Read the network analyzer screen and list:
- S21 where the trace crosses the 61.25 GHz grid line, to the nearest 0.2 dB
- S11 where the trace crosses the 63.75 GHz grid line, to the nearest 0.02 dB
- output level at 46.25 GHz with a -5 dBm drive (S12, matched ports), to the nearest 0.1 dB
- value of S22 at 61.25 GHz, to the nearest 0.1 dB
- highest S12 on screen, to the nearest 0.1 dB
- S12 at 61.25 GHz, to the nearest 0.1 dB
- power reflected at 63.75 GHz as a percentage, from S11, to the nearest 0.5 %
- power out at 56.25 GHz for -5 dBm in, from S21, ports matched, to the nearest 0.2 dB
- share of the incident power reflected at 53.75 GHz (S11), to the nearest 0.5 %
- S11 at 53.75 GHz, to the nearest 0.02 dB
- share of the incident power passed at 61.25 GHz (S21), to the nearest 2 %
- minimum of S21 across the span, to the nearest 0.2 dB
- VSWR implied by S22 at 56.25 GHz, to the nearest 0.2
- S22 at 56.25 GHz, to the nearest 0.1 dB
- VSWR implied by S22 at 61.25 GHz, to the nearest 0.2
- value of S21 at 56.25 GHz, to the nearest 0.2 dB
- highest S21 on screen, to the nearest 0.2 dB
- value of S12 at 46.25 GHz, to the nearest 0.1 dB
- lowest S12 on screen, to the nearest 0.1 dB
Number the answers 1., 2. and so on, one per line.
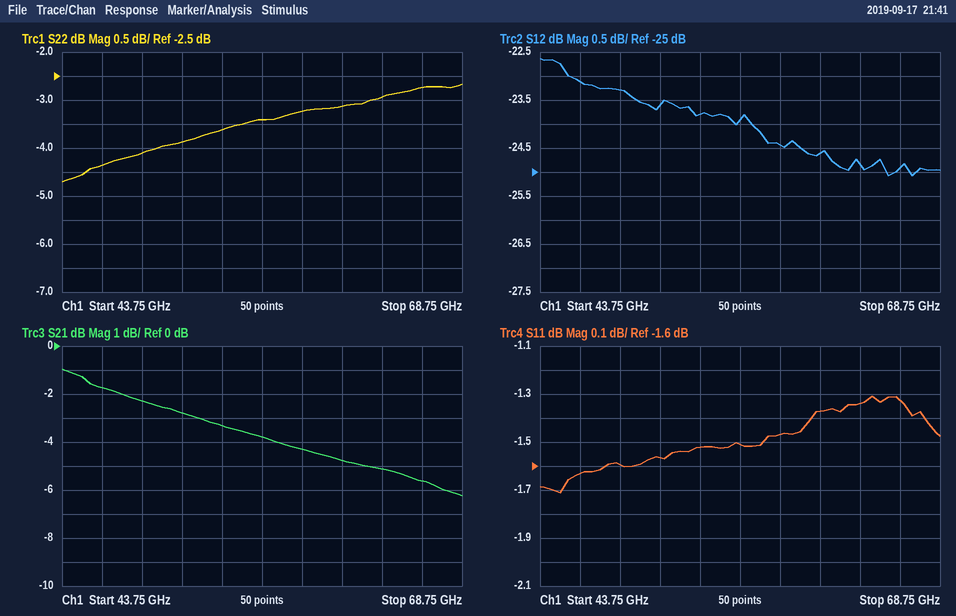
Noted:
1. -4.8 dB
2. -1.34 dB
3. -28.1 dBm
4. -3.1 dB
5. -22.6 dB
6. -24.6 dB
7. 73.5 %
8. -8.8 dBm
9. 70.5 %
10. -1.52 dB
11. 34 %
12. -6.2 dB
13. 5.2
14. -3.4 dB
15. 5.6
16. -3.8 dB
17. -1.0 dB
18. -23.1 dB
19. -25.1 dB
